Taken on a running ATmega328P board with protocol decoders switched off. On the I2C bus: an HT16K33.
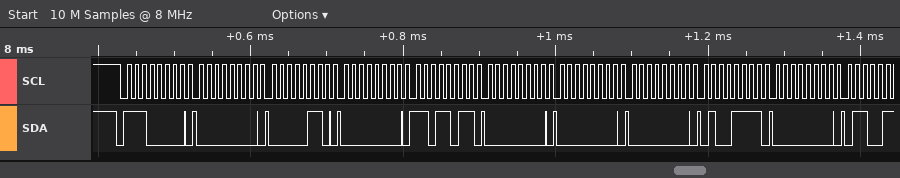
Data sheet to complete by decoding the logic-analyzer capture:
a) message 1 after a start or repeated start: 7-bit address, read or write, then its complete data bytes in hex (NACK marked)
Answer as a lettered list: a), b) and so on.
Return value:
a) 0x70 write: 00 06 00 DB 00 00 00 4F 00
